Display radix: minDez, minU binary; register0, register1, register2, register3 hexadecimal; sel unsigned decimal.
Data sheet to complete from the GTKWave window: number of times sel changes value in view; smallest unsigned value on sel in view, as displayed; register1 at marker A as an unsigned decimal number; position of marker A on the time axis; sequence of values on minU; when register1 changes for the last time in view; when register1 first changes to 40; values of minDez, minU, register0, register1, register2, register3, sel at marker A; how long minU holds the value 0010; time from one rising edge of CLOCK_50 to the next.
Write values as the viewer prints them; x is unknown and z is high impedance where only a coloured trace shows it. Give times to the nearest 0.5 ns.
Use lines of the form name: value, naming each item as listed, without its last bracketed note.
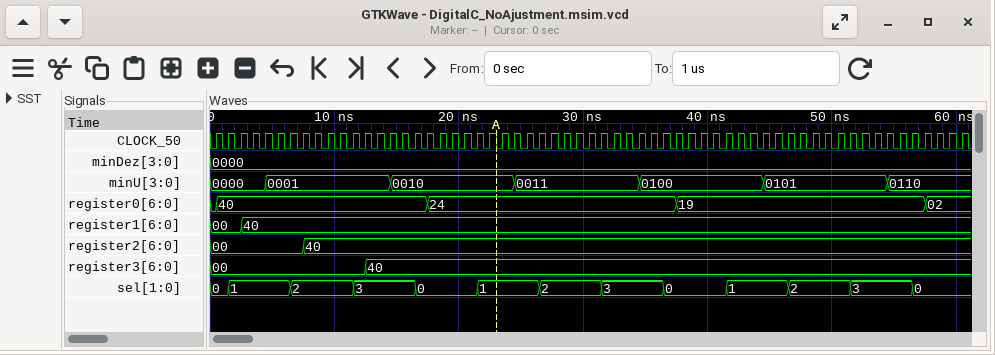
number of times sel changes value in view: 12
smallest unsigned value on sel in view, as displayed: 0
register1 at marker A as an unsigned decimal number: 64
position of marker A on the time axis: 23 ns
sequence of values on minU: 0000, 0001, 0010, 0011, 0100, 0101, 0110
when register1 changes for the last time in view: 2.5 ns
when register1 first changes to 40: 2.5 ns
values of minDez, minU, register0, register1, register2, register3, sel at marker A: minDez=0000, minU=0010, register0=24, register1=40, register2=40, register3=40, sel=1
how long minU holds the value 0010: 10 ns
time from one rising edge of CLOCK_50 to the next: 1 ns
